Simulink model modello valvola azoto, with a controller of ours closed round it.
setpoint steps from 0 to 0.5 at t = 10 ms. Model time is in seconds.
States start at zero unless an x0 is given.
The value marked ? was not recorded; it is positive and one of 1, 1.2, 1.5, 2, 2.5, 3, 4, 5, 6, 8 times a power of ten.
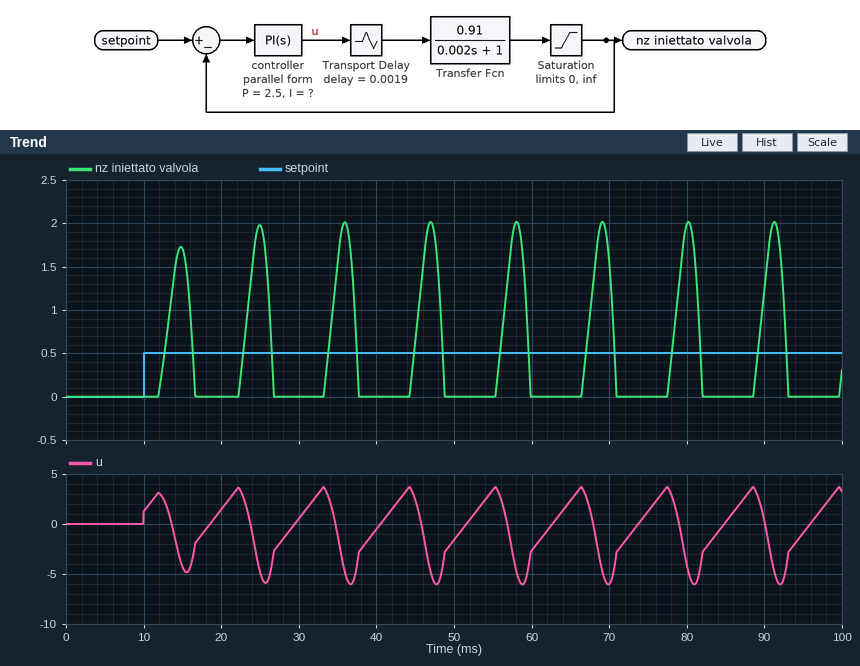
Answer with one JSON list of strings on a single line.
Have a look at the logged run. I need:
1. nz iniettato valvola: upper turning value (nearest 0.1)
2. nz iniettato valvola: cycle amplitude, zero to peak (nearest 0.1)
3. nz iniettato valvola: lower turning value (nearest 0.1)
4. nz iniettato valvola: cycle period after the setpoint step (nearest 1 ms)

["2.0", "1.0", "0.0", "11 ms"]
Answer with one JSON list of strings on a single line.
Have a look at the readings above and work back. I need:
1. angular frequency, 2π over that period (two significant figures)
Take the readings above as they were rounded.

["0.57 rad/ms"]
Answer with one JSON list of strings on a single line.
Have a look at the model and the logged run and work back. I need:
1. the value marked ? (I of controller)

["2000"]
